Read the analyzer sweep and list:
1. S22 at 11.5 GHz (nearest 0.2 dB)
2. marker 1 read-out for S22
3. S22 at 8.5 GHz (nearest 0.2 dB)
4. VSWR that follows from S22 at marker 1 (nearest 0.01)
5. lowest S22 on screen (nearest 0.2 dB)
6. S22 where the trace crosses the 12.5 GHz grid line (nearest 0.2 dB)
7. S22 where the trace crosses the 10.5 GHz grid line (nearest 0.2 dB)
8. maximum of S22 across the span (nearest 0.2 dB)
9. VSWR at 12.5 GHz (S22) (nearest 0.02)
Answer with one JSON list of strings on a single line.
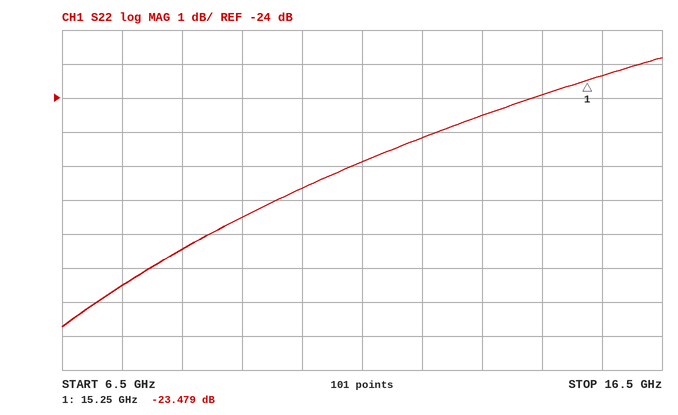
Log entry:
["-25.8 dB", "-23.479 dB", "-28.4 dB", "1.14", "-30.8 dB", "-25.2 dB", "-26.6 dB", "-22.8 dB", "1.12"]
